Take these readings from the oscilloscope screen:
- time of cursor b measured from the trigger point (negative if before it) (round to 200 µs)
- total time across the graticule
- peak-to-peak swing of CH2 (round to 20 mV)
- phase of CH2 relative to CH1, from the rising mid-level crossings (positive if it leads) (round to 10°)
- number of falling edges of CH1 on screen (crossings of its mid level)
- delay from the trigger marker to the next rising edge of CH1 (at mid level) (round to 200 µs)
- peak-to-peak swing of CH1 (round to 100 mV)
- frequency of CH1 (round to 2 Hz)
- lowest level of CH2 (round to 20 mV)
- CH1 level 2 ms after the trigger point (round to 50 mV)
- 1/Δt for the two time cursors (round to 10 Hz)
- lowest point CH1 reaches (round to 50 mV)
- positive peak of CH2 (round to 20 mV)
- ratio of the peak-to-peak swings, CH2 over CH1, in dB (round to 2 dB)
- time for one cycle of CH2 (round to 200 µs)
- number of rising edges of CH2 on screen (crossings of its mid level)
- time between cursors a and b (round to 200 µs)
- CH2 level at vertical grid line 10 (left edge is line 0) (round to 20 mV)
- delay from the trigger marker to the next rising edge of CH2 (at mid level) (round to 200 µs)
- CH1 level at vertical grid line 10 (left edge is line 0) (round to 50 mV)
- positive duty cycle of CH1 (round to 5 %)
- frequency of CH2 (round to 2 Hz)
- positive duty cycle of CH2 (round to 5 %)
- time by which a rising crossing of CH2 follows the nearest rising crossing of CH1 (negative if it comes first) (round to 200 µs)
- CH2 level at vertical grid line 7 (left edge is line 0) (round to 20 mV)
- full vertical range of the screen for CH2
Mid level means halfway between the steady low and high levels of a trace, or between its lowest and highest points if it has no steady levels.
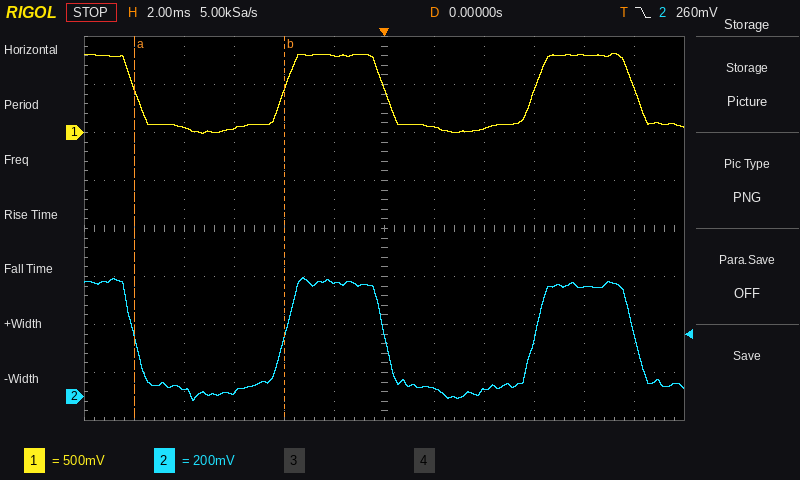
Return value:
-4.0 ms
24 ms
520 mV
0°
3
6.0 ms
800 mV
100 Hz
-20 mV
50 mV
170 Hz
0 mV
500 mV
-4 dB
10.0 ms
2
6.0 ms
460 mV
6.0 ms
800 mV
40 %
100 Hz
40 %
0.0 ms
40 mV
1.6 V
